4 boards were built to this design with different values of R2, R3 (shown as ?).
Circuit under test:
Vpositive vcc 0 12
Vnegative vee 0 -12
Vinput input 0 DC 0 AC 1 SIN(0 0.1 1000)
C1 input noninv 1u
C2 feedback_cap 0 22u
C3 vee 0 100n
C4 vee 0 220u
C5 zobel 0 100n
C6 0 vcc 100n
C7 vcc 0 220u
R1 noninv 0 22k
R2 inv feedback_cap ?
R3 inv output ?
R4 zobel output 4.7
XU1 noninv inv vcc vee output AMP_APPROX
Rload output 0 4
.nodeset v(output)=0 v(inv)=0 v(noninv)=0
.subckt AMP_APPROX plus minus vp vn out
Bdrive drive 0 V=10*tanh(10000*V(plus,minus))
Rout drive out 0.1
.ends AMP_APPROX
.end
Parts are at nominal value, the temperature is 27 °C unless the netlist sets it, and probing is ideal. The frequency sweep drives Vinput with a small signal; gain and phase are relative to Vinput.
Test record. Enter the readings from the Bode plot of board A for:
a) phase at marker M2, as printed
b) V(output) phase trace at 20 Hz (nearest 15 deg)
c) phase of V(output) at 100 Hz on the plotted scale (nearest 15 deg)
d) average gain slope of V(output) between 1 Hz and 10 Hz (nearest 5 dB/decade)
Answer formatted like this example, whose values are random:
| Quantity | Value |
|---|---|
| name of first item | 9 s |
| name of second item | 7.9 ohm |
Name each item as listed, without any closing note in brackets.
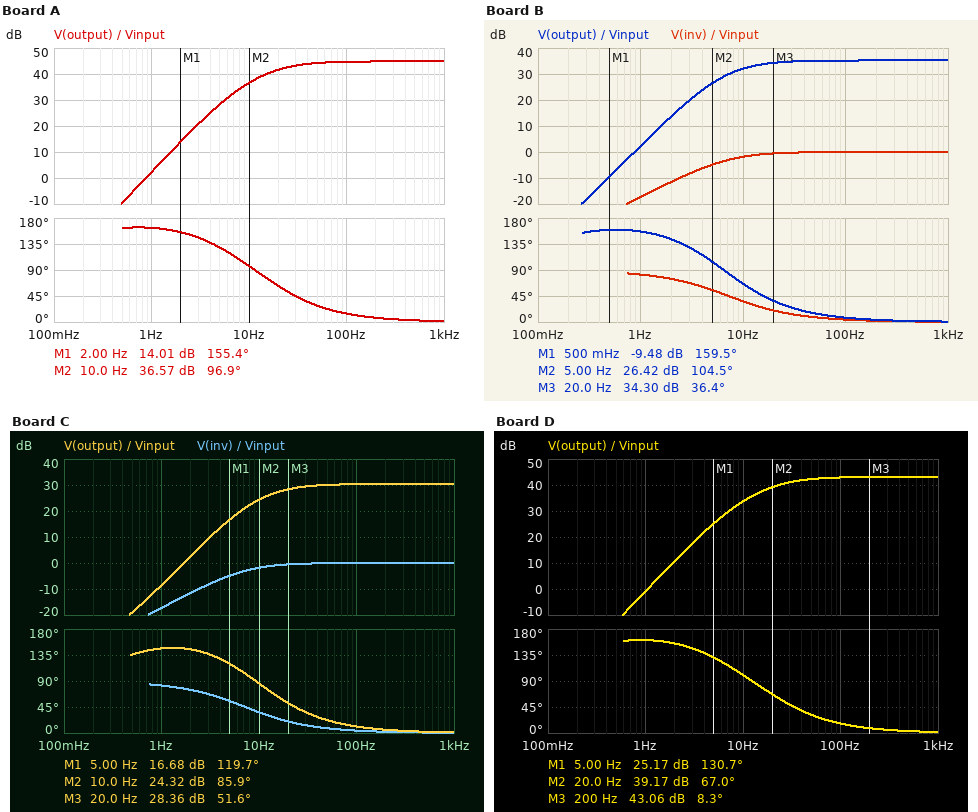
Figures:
| Quantity | Value |
|---|---|
| phase at marker M2, as printed | 96.9 deg |
| V(output) phase trace at 20 Hz | 60 deg |
| phase of V(output) at 100 Hz on the plotted scale | 15 deg |
| average gain slope of V(output) between 1 Hz and 10 Hz | 35 dB/decade |
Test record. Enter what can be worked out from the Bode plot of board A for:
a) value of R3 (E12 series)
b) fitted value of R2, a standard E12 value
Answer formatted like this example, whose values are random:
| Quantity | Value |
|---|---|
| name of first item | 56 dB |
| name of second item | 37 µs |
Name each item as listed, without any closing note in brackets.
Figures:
| Quantity | Value |
|---|---|
| value of R3 | 68 kΩ |
| fitted value of R2, a standard E12 value | 390 Ω |
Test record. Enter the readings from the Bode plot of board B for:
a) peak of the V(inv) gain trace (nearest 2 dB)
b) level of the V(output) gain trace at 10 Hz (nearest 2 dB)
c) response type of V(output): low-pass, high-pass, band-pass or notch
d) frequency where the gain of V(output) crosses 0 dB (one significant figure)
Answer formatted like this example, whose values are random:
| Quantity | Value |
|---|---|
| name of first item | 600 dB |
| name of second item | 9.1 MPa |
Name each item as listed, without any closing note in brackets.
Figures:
| Quantity | Value |
|---|---|
| peak of the V(inv) gain trace | 0 dB |
| level of the V(output) gain trace at 10 Hz | 32 dB |
| response type of V(output): low-pass, high-pass, band-pass or notch | high-pass |
| frequency where the gain of V(output) crosses 0 dB | 900 mHz |
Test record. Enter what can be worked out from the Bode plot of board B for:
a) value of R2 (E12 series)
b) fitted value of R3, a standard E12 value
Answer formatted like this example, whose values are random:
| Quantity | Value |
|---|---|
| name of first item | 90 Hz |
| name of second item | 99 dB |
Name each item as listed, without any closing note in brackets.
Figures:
| Quantity | Value |
|---|---|
| value of R2 | 1.2 kΩ |
| fitted value of R3, a standard E12 value | 68 kΩ |
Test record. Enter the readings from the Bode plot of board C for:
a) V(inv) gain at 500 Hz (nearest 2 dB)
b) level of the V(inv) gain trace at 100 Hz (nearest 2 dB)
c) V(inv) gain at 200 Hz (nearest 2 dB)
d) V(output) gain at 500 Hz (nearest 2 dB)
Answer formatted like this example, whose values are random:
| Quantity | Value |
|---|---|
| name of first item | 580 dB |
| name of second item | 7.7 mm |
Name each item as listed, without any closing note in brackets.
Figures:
| Quantity | Value |
|---|---|
| V(inv) gain at 500 Hz | 0 dB |
| level of the V(inv) gain trace at 100 Hz | 0 dB |
| V(inv) gain at 200 Hz | 0 dB |
| V(output) gain at 500 Hz | 30 dB |
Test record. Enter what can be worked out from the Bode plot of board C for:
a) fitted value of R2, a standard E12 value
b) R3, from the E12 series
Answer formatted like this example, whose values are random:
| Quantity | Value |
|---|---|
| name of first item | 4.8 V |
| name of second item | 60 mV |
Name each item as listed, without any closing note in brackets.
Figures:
| Quantity | Value |
|---|---|
| fitted value of R2, a standard E12 value | 560 Ω |
| R3, from the E12 series | 18 kΩ |
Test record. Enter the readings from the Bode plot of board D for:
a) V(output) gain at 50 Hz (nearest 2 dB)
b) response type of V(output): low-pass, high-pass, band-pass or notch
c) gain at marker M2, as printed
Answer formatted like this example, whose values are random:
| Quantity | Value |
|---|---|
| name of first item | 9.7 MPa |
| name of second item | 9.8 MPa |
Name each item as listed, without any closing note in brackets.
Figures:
| Quantity | Value |
|---|---|
| V(output) gain at 50 Hz | 42 dB |
| response type of V(output): low-pass, high-pass, band-pass or notch | high-pass |
| gain at marker M2, as printed | 39.17 dB |
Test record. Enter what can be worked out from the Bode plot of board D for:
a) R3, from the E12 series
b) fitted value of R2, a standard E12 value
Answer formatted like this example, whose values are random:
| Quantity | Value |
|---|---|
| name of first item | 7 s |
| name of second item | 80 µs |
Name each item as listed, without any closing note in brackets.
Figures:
| Quantity | Value |
|---|---|
| R3, from the E12 series | 47 kΩ |
| fitted value of R2, a standard E12 value | 330 Ω |
